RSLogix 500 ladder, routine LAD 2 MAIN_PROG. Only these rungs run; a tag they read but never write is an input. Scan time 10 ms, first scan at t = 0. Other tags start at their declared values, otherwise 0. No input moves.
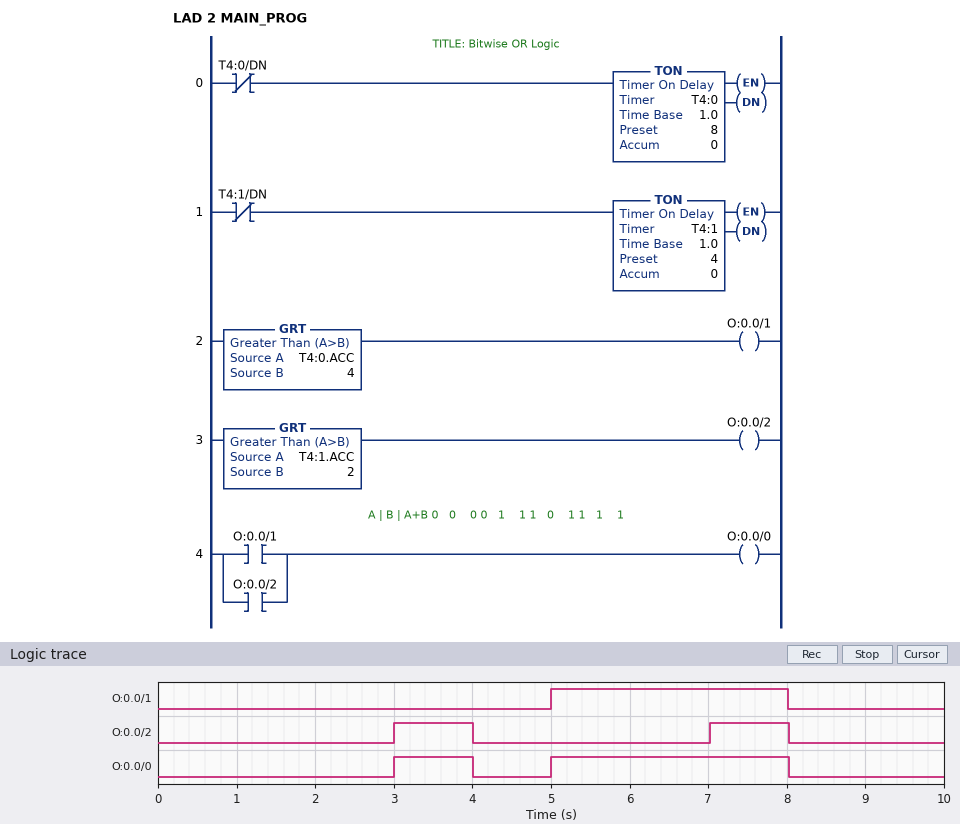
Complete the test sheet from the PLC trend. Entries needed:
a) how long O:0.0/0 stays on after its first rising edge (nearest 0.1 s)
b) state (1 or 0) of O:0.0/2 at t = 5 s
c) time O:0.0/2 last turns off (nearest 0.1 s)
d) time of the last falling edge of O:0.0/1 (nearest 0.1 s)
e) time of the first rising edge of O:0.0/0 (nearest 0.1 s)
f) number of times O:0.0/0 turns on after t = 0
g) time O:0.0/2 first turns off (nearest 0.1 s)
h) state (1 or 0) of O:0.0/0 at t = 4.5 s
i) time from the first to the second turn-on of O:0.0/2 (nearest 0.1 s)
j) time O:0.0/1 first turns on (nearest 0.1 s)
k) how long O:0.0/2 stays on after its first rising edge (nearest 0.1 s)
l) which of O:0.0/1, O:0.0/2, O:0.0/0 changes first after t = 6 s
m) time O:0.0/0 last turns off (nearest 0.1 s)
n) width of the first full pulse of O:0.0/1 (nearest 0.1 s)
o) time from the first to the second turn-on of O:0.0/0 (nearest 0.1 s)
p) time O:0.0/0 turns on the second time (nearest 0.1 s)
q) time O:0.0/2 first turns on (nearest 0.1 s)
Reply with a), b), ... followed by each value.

a) 1.0 s
b) 0
c) 8.0 s
d) 8.0 s
e) 3.0 s
f) 2
g) 4.0 s
h) 0
i) 4.0 s
j) 5.0 s
k) 1.0 s
l) O:0.0/2
m) 8.0 s
n) 3.0 s
o) 2.0 s
p) 5.0 s
q) 3.0 s
